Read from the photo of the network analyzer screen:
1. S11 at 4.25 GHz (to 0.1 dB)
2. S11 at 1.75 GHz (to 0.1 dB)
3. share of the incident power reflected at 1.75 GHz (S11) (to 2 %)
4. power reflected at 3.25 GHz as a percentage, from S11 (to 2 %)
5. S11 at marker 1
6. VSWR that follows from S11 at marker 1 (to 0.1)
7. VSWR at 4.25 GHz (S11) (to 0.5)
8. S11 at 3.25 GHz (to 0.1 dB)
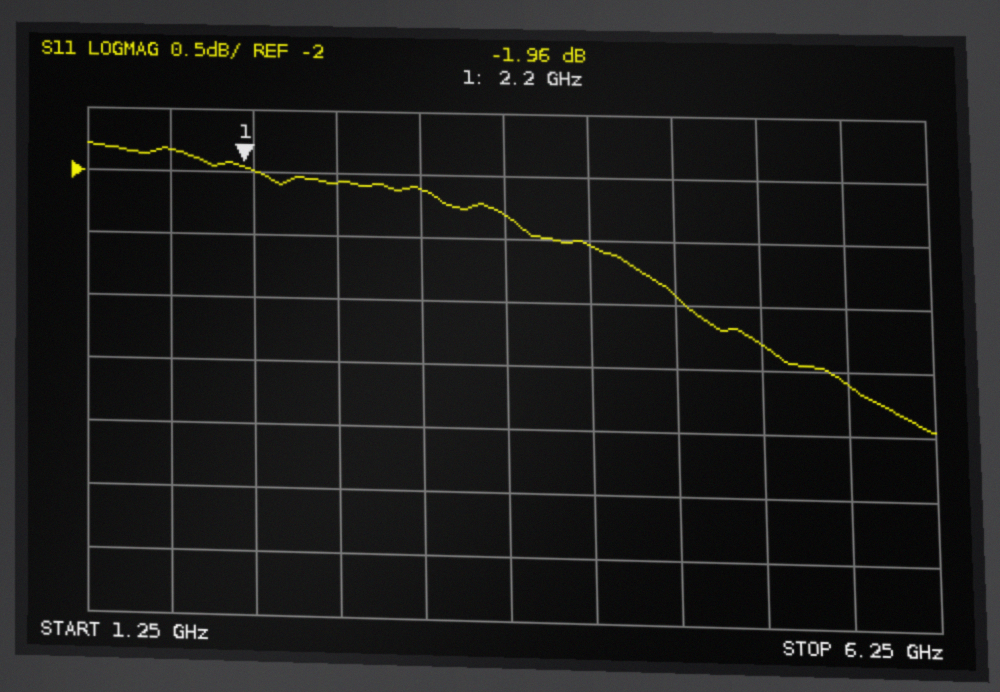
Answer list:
-2.5 dB
-1.8 dB
66 %
62 %
-1.96 dB
8.9
7.0
-2.1 dB
